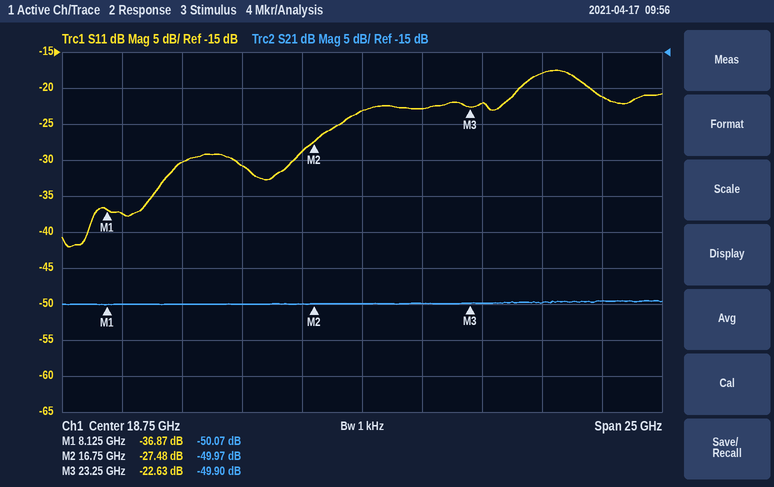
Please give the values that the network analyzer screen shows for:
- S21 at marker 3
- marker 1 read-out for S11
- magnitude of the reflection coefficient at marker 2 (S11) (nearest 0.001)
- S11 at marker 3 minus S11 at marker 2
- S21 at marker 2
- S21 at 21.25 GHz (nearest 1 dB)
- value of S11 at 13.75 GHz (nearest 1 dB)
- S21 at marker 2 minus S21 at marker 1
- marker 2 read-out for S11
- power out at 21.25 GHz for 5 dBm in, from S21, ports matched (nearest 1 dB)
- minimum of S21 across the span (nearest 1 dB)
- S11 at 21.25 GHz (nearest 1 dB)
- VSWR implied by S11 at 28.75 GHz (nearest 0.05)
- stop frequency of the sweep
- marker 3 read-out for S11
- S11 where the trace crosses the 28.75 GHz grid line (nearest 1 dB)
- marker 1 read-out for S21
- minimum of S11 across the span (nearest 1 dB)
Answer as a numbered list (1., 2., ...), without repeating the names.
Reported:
1. -49.90 dB
2. -36.87 dB
3. 0.042
4. 4.85 dB
5. -49.97 dB
6. -50 dB
7. -31 dB
8. 0.10 dB
9. -27.48 dB
10. -45 dBm
11. -50 dB
12. -23 dB
13. 1.20
14. 31.25 GHz
15. -22.63 dB
16. -21 dB
17. -50.07 dB
18. -42 dB
